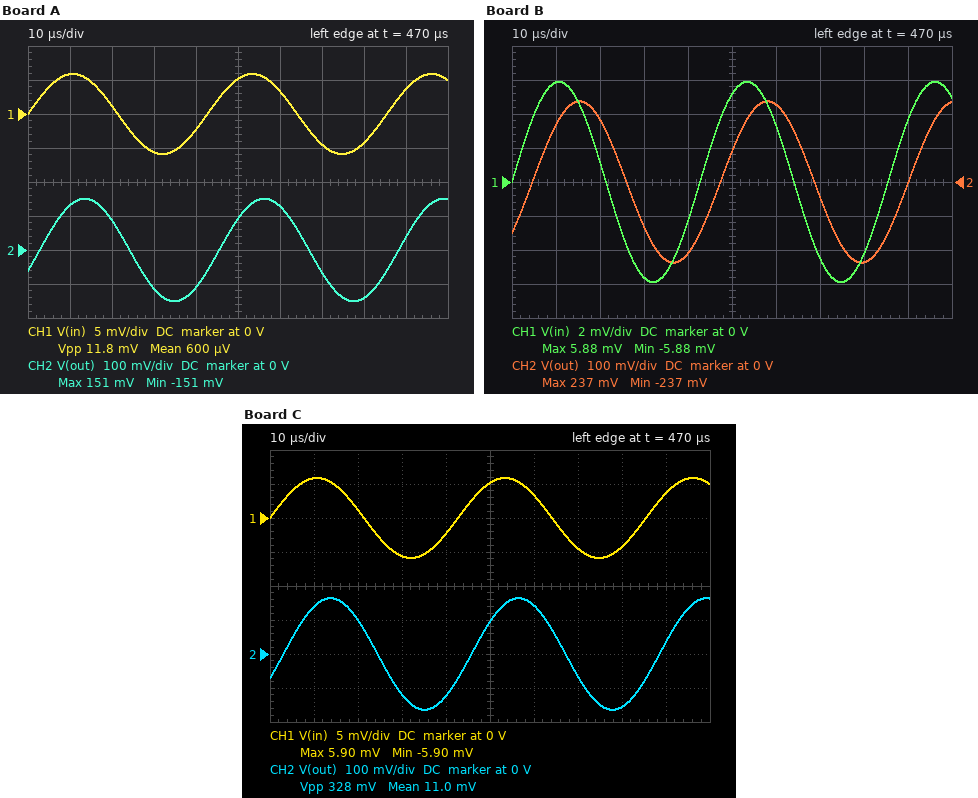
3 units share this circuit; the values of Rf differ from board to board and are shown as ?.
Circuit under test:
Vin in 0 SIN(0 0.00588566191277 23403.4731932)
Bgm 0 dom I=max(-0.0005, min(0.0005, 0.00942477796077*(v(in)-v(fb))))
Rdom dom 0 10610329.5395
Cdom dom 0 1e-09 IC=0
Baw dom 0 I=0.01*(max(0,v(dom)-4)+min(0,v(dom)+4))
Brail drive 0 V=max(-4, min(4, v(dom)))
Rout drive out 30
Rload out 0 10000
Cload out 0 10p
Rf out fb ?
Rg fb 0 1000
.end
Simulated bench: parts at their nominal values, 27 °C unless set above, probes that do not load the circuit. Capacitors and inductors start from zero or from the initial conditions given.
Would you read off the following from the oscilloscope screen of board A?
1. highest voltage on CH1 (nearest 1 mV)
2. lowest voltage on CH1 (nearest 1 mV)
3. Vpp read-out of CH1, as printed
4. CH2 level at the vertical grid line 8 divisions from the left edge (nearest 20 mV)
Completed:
6 mV
-6 mV
11.8 mV
-140 mV
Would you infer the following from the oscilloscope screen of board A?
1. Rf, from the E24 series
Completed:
27 kΩ
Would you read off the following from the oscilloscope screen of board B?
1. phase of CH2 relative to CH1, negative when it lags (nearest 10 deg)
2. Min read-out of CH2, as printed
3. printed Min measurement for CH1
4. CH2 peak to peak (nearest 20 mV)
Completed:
-40 deg
-237 mV
-5.88 mV
480 mV
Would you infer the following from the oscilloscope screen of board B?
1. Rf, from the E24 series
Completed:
51 kΩ
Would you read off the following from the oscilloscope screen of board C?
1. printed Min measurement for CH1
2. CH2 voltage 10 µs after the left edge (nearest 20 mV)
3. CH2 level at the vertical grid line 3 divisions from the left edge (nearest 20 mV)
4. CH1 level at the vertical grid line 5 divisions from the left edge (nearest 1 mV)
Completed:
-5.90 mV
140 mV
-120 mV
5 mV
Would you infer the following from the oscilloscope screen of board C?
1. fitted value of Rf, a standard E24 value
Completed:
30 kΩ
